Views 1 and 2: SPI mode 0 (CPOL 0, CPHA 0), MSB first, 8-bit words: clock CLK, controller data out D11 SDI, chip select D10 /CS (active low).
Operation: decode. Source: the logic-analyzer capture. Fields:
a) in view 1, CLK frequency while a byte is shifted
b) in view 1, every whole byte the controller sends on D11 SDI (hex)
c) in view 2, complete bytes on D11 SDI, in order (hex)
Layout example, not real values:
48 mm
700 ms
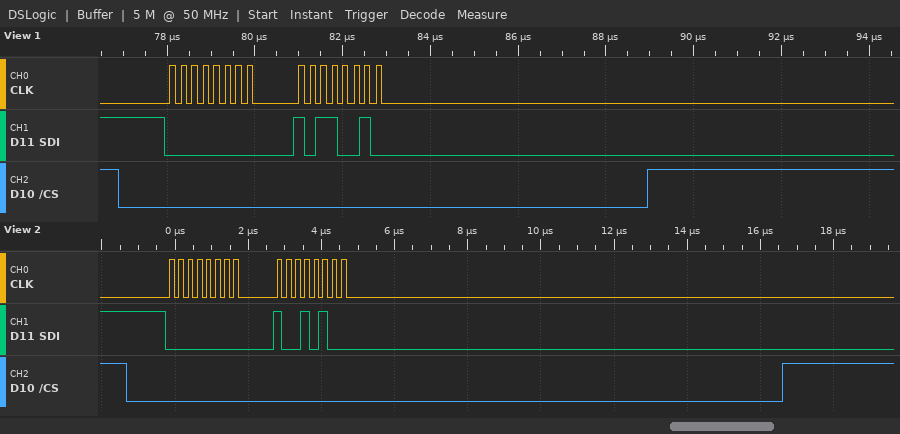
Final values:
4 MHz
00 B2
00 94
